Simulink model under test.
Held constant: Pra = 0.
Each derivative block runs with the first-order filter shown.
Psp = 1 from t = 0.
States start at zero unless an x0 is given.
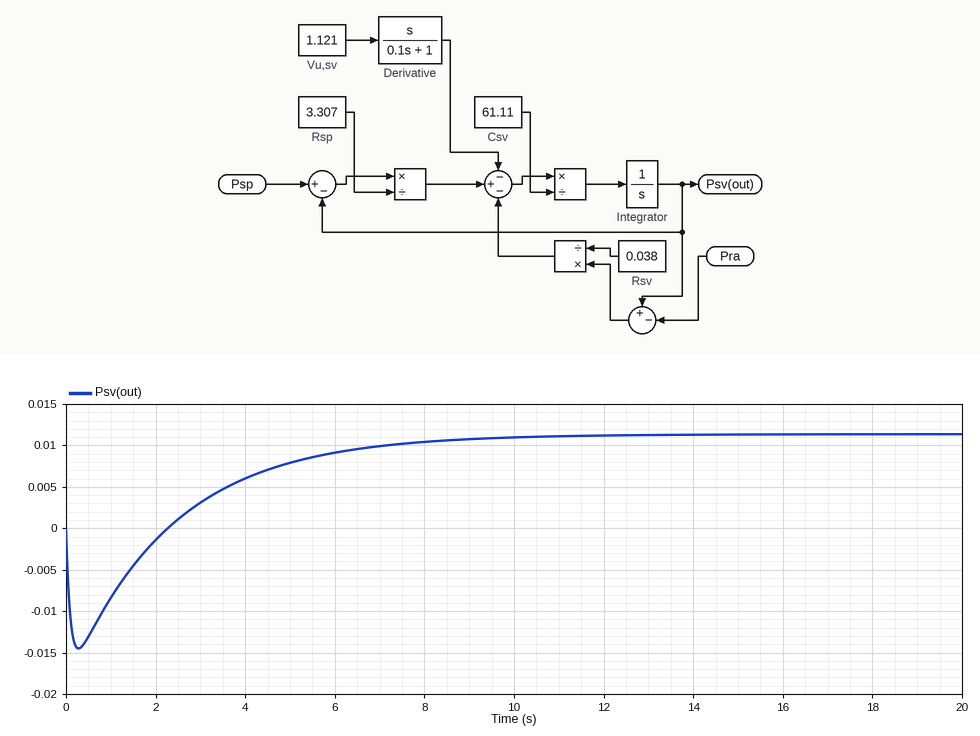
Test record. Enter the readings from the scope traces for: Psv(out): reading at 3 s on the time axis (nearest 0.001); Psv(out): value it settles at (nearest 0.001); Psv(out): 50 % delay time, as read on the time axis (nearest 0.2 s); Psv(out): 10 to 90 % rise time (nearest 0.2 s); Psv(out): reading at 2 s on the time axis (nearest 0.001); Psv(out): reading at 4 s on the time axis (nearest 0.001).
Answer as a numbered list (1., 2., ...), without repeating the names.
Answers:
1. 0.003
2. 0.011
3. 3.8 s
4. 5.0 s
5. -0.001
6. 0.006
